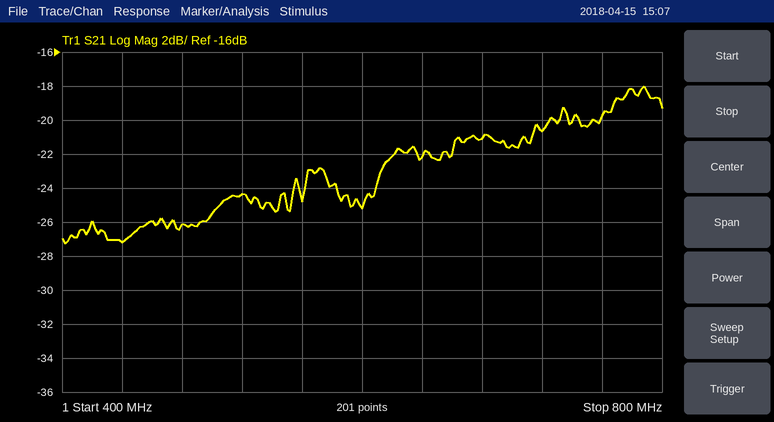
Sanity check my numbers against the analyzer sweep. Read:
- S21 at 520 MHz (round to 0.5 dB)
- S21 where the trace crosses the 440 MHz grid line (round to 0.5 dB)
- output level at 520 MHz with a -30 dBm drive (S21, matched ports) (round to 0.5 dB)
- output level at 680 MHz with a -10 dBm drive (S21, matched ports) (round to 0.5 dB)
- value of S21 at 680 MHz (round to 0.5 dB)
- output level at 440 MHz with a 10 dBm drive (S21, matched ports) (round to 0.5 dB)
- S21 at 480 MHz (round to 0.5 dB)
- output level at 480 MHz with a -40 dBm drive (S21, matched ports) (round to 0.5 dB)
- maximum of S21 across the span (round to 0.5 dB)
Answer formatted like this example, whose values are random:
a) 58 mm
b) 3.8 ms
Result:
a) -24.5 dB
b) -27.0 dB
c) -54.5 dBm
d) -31.0 dBm
e) -21.0 dB
f) -17.0 dBm
g) -26.0 dB
h) -66.0 dBm
i) -18.0 dB
